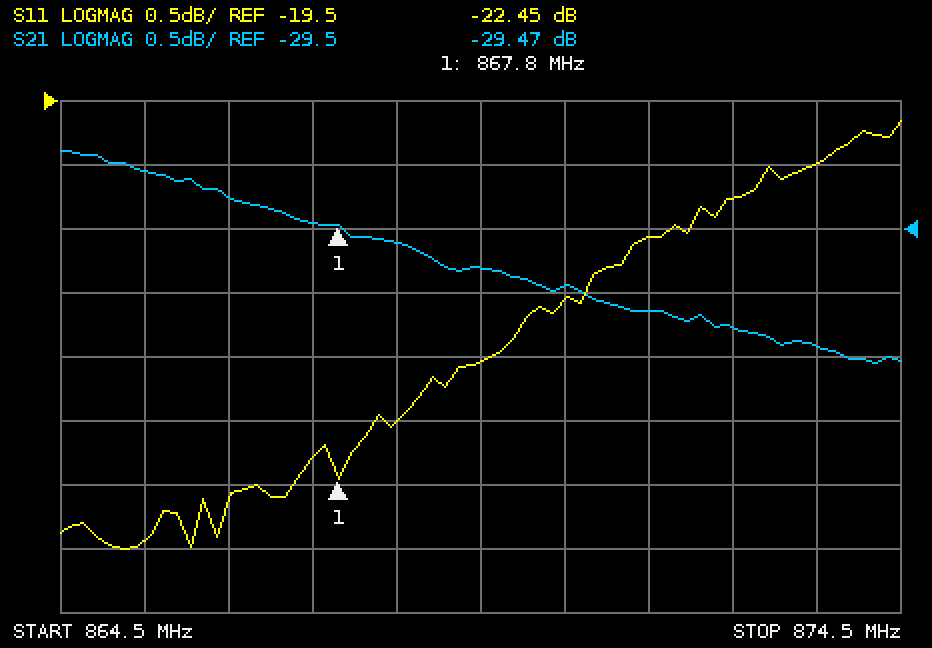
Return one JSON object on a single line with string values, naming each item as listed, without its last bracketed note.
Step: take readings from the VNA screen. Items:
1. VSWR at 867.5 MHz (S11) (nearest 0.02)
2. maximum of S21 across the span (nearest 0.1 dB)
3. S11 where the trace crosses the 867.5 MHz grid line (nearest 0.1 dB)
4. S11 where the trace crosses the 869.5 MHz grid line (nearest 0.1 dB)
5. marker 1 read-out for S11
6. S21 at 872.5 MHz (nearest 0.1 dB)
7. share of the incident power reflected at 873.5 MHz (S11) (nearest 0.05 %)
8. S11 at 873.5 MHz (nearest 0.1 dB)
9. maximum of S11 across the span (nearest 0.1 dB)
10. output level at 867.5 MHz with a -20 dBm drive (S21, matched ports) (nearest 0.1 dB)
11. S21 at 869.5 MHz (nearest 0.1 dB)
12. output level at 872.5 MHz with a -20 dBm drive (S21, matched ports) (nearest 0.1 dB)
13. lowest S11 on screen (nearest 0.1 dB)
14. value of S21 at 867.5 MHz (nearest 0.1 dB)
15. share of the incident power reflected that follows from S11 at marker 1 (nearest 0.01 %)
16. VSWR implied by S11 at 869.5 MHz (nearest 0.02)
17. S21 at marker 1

{"VSWR at 867.5 MHz (S11)": "1.16", "maximum of S21 across the span": "-28.9 dB", "S11 where the trace crosses the 867.5 MHz grid line": "-22.3 dB", "S11 where the trace crosses the 869.5 MHz grid line": "-21.5 dB", "marker 1 read-out for S11": "-22.45 dB", "S21 at 872.5 MHz": "-30.3 dB", "share of the incident power reflected at 873.5 MHz (S11)": "1.00 %", "S11 at 873.5 MHz": "-20.0 dB", "maximum of S11 across the span": "-19.7 dB", "output level at 867.5 MHz with a -20 dBm drive (S21, matched ports)": "-49.5 dBm", "S21 at 869.5 MHz": "-29.8 dB", "output level at 872.5 MHz with a -20 dBm drive (S21, matched ports)": "-50.3 dBm", "lowest S11 on screen": "-23.0 dB", "value of S21 at 867.5 MHz": "-29.5 dB", "share of the incident power reflected that follows from S11 at marker 1": "0.57 %", "VSWR implied by S11 at 869.5 MHz": "1.18", "S21 at marker 1": "-29.47 dB"}
